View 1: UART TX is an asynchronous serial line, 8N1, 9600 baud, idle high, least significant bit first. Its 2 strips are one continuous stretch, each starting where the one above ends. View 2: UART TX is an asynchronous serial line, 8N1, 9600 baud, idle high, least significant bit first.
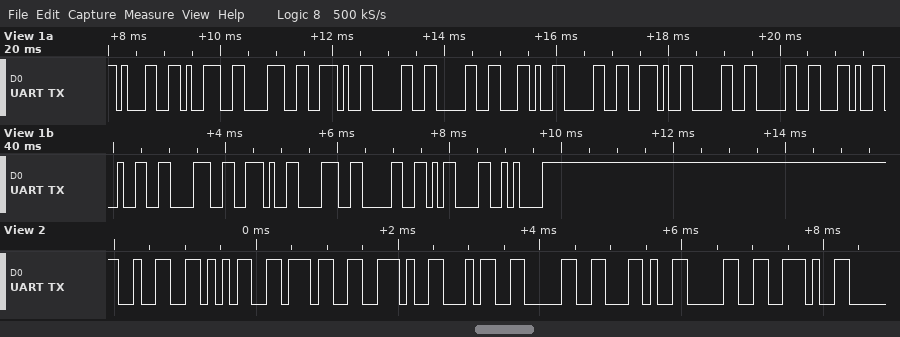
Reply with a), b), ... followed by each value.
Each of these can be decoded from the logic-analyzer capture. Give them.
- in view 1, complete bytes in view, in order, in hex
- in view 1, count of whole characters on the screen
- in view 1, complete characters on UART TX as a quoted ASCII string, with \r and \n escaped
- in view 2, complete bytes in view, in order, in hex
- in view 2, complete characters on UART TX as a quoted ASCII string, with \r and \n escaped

a) 31 39 38 2E 30 30 2C 30 2E 30 30 2C 32 38 2E 38 30 0D 0A
b) 19
c) "198.00,0.00,28.80\r\n"
d) 32 35 37 2E 34 30 2C 30 2E
e) "257.40,0."
